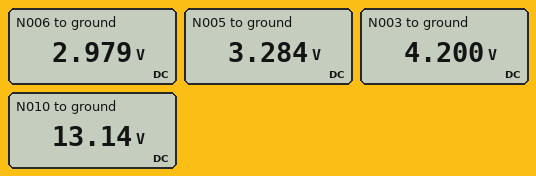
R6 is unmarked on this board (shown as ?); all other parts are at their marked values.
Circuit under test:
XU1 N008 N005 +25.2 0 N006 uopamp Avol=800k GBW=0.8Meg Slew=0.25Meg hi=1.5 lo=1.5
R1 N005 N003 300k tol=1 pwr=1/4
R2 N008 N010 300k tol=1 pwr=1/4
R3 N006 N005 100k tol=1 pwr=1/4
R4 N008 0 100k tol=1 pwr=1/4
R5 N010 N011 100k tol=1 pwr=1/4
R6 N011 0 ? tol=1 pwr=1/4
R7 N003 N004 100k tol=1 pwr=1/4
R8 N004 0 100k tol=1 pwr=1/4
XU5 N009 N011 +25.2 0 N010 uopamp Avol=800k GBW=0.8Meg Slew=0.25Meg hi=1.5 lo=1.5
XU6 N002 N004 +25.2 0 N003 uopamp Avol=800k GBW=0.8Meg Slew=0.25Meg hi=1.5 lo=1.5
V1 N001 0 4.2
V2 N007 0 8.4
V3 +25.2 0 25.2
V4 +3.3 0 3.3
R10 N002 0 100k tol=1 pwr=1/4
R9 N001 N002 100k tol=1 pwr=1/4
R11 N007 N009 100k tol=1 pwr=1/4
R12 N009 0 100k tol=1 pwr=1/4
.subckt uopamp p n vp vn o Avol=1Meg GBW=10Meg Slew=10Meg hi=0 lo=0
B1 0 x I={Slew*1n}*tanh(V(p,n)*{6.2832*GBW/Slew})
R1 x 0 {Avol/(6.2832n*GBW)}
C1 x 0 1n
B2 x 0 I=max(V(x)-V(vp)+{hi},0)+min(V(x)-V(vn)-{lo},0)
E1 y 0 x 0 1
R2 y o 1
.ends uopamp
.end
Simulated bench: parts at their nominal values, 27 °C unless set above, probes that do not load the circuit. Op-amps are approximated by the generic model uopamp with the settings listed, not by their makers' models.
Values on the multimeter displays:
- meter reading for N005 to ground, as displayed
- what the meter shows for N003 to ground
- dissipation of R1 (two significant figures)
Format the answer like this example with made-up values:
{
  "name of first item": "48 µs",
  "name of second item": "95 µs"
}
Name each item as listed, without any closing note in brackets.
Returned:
{
  "meter reading for N005 to ground, as displayed": "3.284 V",
  "what the meter shows for N003 to ground": "4.200 V",
  "dissipation of R1": "2.8 µW"
}
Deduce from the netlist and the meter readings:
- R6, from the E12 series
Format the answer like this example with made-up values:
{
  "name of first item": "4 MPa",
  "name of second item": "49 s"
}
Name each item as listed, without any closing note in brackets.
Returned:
{
  "R6, from the E12 series": "47 kΩ"
}
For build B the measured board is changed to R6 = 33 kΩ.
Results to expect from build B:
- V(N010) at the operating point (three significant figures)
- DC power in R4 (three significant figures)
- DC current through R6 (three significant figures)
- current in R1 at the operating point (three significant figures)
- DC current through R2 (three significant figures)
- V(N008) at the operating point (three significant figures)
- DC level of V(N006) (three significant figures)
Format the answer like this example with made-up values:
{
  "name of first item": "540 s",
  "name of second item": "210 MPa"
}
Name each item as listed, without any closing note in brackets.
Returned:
{
  "V(N010) at the operating point": "16.9 V",
  "DC power in R4": "179 µW",
  "DC current through R6": "127 µA",
  "current in R1 at the operating point": "106 nA",
  "DC current through R2": "42.3 µA",
  "V(N008) at the operating point": "4.23 V",
  "DC level of V(N006)": "4.24 V"
}
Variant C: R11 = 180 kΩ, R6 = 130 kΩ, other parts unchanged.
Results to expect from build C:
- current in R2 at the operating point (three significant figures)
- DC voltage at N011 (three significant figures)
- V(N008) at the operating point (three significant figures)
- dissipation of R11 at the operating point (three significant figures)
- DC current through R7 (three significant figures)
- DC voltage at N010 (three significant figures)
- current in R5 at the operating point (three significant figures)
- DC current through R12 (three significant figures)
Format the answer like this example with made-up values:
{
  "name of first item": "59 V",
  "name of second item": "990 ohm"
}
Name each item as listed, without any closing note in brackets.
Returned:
{
  "current in R2 at the operating point": "13.3 µA",
  "DC voltage at N011": "3.00 V",
  "V(N008) at the operating point": "1.33 V",
  "dissipation of R11 at the operating point": "162 µW",
  "DC current through R7": "21.0 µA",
  "DC voltage at N010": "5.31 V",
  "current in R5 at the operating point": "23.1 µA",
  "DC current through R12": "30.0 µA"
}
